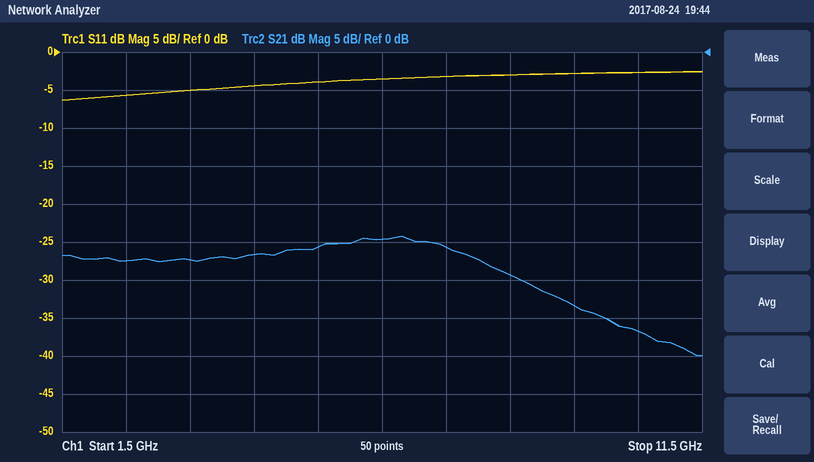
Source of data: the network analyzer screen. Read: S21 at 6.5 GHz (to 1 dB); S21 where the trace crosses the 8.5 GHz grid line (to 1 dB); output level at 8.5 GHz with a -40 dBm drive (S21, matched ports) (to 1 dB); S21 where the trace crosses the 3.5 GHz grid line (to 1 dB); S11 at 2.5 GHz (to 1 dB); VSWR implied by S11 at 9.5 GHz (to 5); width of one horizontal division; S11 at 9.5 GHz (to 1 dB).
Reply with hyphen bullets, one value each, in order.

- -25 dB
- -29 dB
- -69 dBm
- -27 dB
- -6 dB
- 5
- 1 GHz
- -3 dB
